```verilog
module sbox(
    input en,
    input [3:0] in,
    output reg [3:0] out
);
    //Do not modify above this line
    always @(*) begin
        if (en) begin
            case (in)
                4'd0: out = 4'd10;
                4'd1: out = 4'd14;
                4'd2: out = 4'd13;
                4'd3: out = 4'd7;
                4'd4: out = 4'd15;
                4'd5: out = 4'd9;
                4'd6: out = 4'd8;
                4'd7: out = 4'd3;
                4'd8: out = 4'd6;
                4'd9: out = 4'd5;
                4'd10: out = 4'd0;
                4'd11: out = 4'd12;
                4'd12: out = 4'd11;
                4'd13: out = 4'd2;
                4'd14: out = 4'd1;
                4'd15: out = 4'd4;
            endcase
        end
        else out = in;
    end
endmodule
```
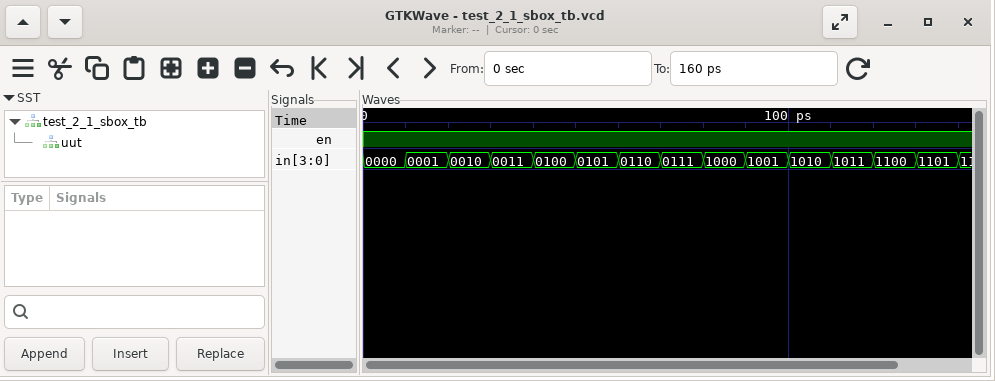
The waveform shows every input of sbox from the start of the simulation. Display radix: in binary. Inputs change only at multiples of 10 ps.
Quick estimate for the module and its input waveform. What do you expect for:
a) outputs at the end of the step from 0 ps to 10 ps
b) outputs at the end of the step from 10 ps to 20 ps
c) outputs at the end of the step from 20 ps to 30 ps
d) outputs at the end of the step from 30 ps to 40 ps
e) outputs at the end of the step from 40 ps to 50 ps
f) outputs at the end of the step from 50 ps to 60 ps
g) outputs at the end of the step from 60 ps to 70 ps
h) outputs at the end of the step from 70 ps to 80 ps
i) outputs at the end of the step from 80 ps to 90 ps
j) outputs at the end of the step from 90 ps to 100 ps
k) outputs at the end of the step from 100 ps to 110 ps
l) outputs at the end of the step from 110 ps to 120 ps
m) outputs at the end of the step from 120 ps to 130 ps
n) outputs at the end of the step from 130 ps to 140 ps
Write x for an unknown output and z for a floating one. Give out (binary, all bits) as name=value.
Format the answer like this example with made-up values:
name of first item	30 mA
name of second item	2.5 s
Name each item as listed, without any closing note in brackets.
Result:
outputs at the end of the step from 0 ps to 10 ps	out=1010
outputs at the end of the step from 10 ps to 20 ps	out=1110
outputs at the end of the step from 20 ps to 30 ps	out=1101
outputs at the end of the step from 30 ps to 40 ps	out=0111
outputs at the end of the step from 40 ps to 50 ps	out=1111
outputs at the end of the step from 50 ps to 60 ps	out=1001
outputs at the end of the step from 60 ps to 70 ps	out=1000
outputs at the end of the step from 70 ps to 80 ps	out=0011
outputs at the end of the step from 80 ps to 90 ps	out=0110
outputs at the end of the step from 90 ps to 100 ps	out=0101
outputs at the end of the step from 100 ps to 110 ps	out=0000
outputs at the end of the step from 110 ps to 120 ps	out=1100
outputs at the end of the step from 120 ps to 130 ps	out=1011
outputs at the end of the step from 130 ps to 140 ps	out=0010
